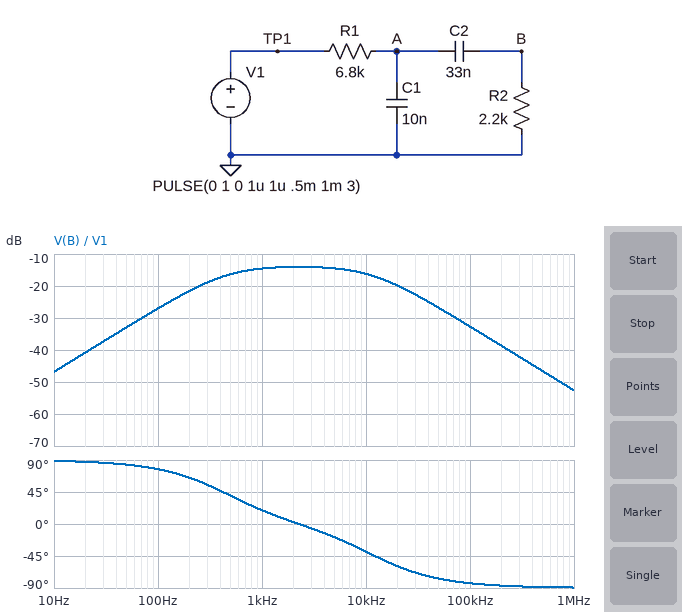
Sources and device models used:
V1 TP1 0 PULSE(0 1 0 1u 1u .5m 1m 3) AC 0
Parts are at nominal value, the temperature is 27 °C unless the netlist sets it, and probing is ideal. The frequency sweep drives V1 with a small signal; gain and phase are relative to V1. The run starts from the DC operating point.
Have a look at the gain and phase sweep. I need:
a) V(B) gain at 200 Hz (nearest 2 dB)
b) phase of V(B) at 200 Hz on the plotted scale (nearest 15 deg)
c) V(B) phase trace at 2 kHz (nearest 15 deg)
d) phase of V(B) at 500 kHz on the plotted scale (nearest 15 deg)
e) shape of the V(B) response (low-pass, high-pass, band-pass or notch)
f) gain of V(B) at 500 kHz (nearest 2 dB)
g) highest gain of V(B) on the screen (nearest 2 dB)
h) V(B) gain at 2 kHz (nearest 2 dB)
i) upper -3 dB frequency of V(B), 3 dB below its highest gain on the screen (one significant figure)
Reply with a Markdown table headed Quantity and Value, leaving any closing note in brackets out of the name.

| Quantity | Value |
|---|---|
| V(B) gain at 200 Hz | -22 dB |
| phase of V(B) at 200 Hz on the plotted scale | 60 deg |
| V(B) phase trace at 2 kHz | 0 deg |
| phase of V(B) at 500 kHz on the plotted scale | -90 deg |
| shape of the V(B) response | band-pass |
| gain of V(B) at 500 kHz | -46 dB |
| highest gain of V(B) on the screen | -14 dB |
| V(B) gain at 2 kHz | -14 dB |
| upper -3 dB frequency of V(B), 3 dB below its highest gain on the screen | 10 kHz |
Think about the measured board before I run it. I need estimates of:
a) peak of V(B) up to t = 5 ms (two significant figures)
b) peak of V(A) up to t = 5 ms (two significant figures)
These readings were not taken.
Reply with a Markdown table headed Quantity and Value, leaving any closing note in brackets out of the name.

| Quantity | Value |
|---|---|
| peak of V(B) up to t = 5 ms | 180 mV |
| peak of V(A) up to t = 5 ms | 840 mV |
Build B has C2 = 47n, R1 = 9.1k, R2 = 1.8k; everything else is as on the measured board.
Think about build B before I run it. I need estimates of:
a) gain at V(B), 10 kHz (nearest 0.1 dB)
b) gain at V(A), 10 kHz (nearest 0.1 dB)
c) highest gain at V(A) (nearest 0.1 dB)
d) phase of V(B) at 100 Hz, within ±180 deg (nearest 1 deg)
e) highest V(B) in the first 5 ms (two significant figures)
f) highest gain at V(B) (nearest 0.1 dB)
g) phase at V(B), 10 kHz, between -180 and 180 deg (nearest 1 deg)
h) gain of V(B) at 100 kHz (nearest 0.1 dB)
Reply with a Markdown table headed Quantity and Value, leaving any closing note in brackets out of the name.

| Quantity | Value |
|---|---|
| gain at V(B), 10 kHz | -19.1 dB |
| gain at V(A), 10 kHz | -19.0 dB |
| highest gain at V(A) | 0 dB |
| phase of V(B) at 100 Hz, within ±180 deg | 69 deg |
| highest V(B) in the first 5 ms | 130 mV |
| highest gain at V(B) | -17.1 dB |
| phase at V(B), 10 kHz, between -180 and 180 deg | -38 deg |
| gain of V(B) at 100 kHz | -35.2 dB |
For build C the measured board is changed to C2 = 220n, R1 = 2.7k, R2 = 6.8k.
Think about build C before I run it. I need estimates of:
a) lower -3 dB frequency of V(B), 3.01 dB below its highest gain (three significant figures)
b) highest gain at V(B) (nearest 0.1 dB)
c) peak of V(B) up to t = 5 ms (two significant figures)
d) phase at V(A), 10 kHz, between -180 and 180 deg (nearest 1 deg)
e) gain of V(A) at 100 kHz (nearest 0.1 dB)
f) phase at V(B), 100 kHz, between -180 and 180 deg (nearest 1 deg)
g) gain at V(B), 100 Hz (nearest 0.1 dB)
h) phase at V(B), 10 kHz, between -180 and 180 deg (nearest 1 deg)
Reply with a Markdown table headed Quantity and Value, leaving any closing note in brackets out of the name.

| Quantity | Value |
|---|---|
| lower -3 dB frequency of V(B), 3.01 dB below its highest gain | 74.5 Hz |
| highest gain at V(B) | -3.0 dB |
| peak of V(B) up to t = 5 ms | 680 mV |
| phase at V(A), 10 kHz, between -180 and 180 deg | -51 deg |
| gain of V(A) at 100 kHz | -24.6 dB |
| phase at V(B), 100 kHz, between -180 and 180 deg | -85 deg |
| gain at V(B), 100 Hz | -4.9 dB |
| phase at V(B), 10 kHz, between -180 and 180 deg | -50 deg |
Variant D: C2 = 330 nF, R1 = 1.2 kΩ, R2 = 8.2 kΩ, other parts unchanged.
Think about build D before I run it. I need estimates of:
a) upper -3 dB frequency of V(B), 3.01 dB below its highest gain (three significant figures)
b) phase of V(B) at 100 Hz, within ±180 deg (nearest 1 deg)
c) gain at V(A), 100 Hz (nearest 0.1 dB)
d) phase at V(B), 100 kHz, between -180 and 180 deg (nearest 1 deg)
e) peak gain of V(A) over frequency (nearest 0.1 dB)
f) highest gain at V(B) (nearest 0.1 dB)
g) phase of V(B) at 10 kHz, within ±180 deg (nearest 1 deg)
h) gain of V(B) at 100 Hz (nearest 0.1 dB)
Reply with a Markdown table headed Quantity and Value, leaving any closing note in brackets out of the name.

| Quantity | Value |
|---|---|
| upper -3 dB frequency of V(B), 3.01 dB below its highest gain | 15.3 kHz |
| phase of V(B) at 100 Hz, within ±180 deg | 27 deg |
| gain at V(A), 100 Hz | -0.9 dB |
| phase at V(B), 100 kHz, between -180 and 180 deg | -81 deg |
| peak gain of V(A) over frequency | 0 dB |
| highest gain at V(B) | -1.2 dB |
| phase of V(B) at 10 kHz, within ±180 deg | -33 deg |
| gain of V(B) at 100 Hz | -2.2 dB |
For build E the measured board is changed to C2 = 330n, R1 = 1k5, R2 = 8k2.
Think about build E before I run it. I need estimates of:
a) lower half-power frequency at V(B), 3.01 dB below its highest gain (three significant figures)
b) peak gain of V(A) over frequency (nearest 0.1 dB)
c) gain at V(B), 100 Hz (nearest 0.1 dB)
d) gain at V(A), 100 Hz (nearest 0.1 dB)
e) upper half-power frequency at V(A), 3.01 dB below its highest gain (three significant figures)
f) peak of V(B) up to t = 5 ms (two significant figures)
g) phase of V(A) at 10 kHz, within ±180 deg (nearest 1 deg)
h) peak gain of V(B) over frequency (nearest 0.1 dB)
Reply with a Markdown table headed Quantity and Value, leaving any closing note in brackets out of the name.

| Quantity | Value |
|---|---|
| lower half-power frequency at V(B), 3.01 dB below its highest gain | 49.3 Hz |
| peak gain of V(A) over frequency | 0 dB |
| gain at V(B), 100 Hz | -2.4 dB |
| gain at V(A), 100 Hz | -1.1 dB |
| upper half-power frequency at V(A), 3.01 dB below its highest gain | 8.21 kHz |
| peak of V(B) up to t = 5 ms | 830 mV |
| phase of V(A) at 10 kHz, within ±180 deg | -39 deg |
| peak gain of V(B) over frequency | -1.5 dB |
